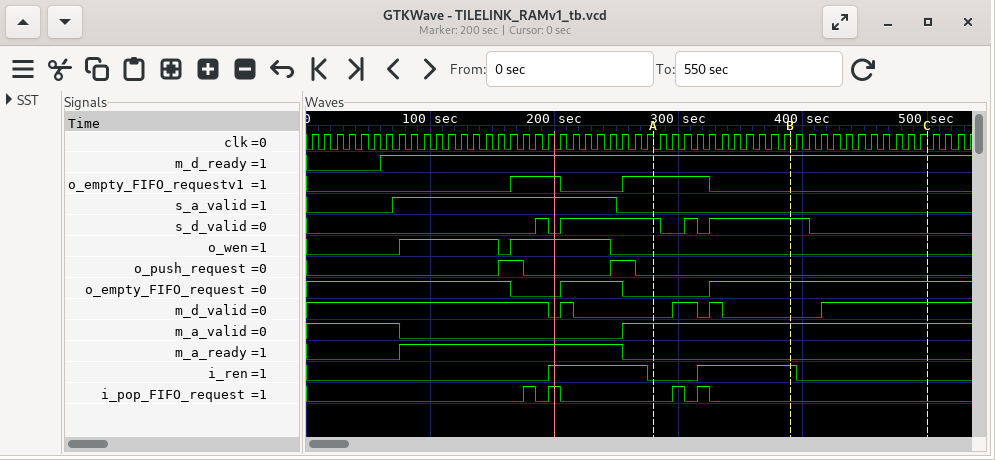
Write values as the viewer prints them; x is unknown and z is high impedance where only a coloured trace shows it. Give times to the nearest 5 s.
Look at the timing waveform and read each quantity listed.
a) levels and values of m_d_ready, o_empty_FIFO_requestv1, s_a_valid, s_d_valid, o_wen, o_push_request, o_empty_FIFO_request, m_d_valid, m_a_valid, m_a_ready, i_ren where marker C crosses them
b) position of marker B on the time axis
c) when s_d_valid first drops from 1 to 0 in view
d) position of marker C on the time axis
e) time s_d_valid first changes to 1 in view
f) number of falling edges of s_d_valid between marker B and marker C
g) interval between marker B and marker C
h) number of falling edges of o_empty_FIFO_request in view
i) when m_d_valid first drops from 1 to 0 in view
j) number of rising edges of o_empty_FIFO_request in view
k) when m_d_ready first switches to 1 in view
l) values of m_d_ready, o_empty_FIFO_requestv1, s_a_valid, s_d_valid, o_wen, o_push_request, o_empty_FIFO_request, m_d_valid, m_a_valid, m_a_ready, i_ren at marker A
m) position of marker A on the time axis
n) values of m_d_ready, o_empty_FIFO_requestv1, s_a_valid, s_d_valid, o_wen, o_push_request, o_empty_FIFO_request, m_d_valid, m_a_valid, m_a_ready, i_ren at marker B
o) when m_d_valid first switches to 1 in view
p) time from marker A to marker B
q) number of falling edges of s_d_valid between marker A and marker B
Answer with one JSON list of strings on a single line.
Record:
["m_d_ready=1, o_empty_FIFO_requestv1=0, s_a_valid=0, s_d_valid=0, o_wen=0, o_push_request=0, o_empty_FIFO_request=1, m_d_valid=1, m_a_valid=1, m_a_ready=0, i_ren=0", "390 s", "195 s", "500 s", "185 s", "1", "110 s", "2", "195 s", "2", "60 s", "m_d_ready=1, o_empty_FIFO_requestv1=1, s_a_valid=0, s_d_valid=1, o_wen=0, o_push_request=0, o_empty_FIFO_request=0, m_d_valid=0, m_a_valid=1, m_a_ready=0, i_ren=0", "280 s", "m_d_ready=1, o_empty_FIFO_requestv1=0, s_a_valid=0, s_d_valid=1, o_wen=0, o_push_request=0, o_empty_FIFO_request=1, m_d_valid=0, m_a_valid=1, m_a_ready=0, i_ren=1", "205 s", "110 s", "2"]
